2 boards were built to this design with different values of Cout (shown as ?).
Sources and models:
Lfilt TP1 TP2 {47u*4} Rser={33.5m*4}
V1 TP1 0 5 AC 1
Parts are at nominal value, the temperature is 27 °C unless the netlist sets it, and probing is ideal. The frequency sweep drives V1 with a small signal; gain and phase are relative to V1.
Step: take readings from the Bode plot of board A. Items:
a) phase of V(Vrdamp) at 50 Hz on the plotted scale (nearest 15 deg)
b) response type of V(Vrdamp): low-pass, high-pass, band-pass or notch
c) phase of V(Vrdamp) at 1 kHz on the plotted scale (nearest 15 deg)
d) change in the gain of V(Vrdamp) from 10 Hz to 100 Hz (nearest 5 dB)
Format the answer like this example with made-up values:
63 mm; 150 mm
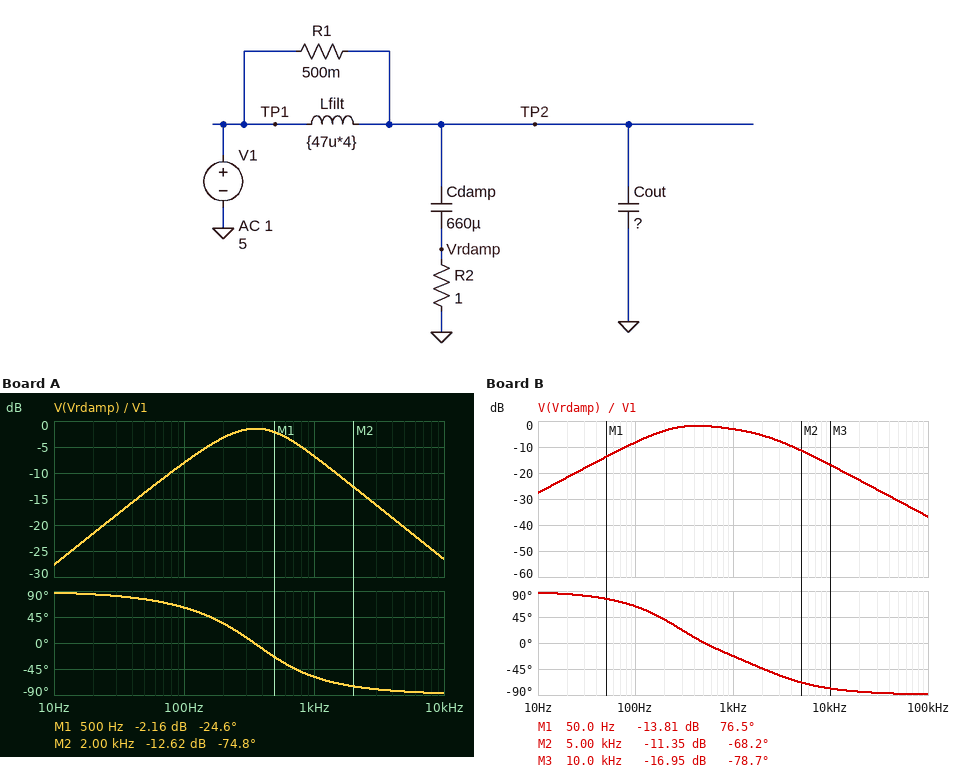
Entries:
75 deg; band-pass; -60 deg; 20 dB
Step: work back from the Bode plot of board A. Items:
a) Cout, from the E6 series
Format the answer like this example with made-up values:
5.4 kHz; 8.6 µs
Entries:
680 µF
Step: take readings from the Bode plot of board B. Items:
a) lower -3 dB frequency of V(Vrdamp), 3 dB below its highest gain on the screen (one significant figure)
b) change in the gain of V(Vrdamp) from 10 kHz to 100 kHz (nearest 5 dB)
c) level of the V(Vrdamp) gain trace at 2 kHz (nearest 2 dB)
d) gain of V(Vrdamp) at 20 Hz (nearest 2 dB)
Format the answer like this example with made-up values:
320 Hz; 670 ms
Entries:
200 Hz; -20 dB; -6 dB; -22 dB
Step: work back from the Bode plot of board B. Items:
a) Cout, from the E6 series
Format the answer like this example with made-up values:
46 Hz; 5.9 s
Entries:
220 µF
